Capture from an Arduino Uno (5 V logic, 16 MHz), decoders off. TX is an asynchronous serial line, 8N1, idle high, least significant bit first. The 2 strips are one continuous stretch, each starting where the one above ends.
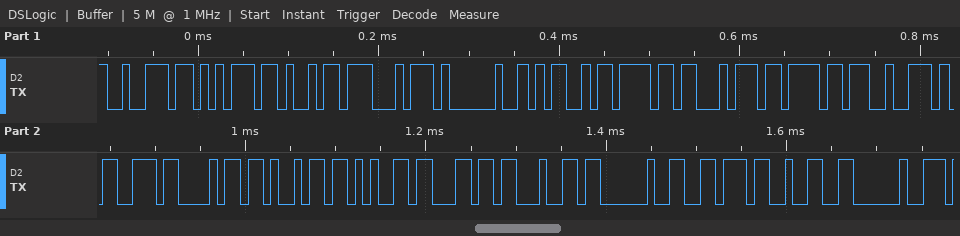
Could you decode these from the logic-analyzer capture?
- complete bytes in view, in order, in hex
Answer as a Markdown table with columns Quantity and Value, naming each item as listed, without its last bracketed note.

| Quantity | Value |
|---|---|
| complete bytes in view, in order, in hex | 72 75 69 74 20 4D 6F 74 6F 72 73 68 69 65 6C 64 20 76 32 20 |
